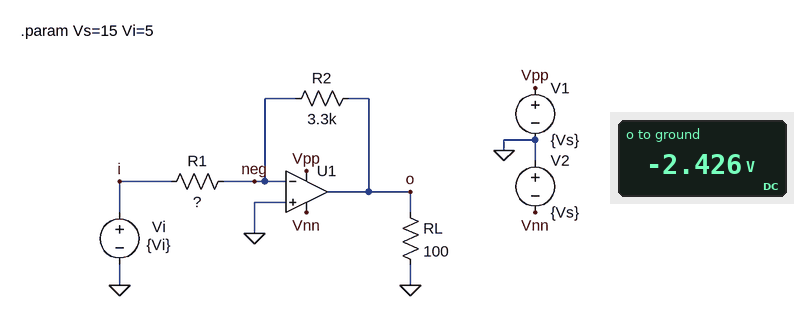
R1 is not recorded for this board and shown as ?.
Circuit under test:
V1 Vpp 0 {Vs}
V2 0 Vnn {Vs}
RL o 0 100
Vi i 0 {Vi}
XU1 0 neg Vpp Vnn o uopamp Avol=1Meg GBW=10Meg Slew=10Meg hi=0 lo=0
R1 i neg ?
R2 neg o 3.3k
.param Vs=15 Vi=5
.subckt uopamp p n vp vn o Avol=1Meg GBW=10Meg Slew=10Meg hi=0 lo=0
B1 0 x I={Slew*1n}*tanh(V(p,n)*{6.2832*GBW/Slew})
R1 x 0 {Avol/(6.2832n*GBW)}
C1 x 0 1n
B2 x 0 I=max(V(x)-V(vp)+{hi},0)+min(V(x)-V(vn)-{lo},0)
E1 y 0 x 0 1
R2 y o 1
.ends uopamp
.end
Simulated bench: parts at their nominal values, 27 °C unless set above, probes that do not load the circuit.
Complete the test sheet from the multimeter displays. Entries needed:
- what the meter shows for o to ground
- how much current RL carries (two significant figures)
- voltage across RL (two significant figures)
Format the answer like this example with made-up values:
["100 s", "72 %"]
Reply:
["-2.426 V", "24 mA", "2.4 V"]
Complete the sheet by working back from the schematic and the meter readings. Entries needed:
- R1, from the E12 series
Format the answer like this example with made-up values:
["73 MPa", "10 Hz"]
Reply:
["6.8 kΩ"]
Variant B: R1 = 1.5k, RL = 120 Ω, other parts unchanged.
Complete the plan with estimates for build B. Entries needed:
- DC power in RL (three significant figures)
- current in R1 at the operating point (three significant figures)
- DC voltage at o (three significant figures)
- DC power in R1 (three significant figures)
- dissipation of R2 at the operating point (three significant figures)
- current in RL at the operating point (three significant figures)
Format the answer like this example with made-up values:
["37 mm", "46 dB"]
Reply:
["1.01 W", "3.33 mA", "-11.0 V", "16.7 mW", "36.7 mW", "91.7 mA"]
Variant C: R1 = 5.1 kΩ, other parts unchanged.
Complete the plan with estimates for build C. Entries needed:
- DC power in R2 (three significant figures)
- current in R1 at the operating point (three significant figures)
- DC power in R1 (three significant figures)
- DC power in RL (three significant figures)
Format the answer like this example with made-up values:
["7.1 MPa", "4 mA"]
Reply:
["3.17 mW", "980 µA", "4.90 mW", "105 mW"]
